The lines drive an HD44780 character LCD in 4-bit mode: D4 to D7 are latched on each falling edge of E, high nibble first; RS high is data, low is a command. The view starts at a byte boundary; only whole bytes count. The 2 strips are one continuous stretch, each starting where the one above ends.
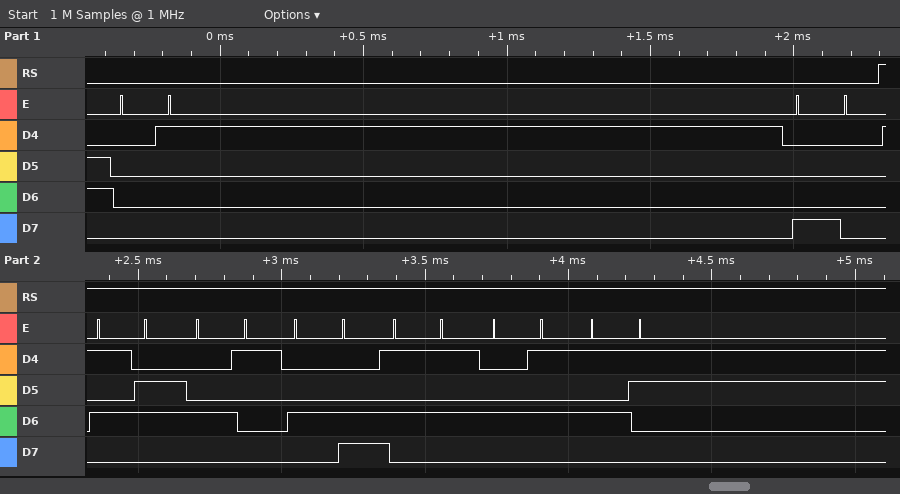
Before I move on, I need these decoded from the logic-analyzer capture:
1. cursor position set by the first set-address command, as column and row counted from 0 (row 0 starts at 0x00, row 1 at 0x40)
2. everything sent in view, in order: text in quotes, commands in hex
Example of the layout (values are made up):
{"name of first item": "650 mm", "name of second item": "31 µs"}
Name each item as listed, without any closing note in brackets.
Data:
{"cursor position set by the first set-address command, as column and row counted from 0": "column 0, row 0", "everything sent in view, in order: text in quotes, commands in hex": "0x01 0x80 \"VALUES\""}
